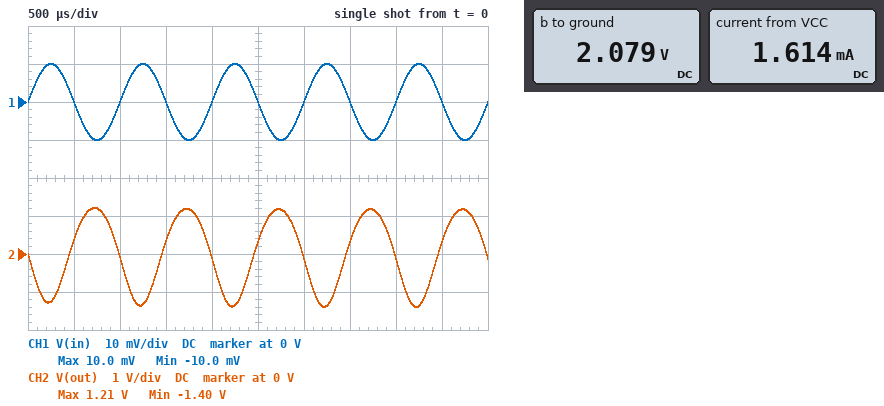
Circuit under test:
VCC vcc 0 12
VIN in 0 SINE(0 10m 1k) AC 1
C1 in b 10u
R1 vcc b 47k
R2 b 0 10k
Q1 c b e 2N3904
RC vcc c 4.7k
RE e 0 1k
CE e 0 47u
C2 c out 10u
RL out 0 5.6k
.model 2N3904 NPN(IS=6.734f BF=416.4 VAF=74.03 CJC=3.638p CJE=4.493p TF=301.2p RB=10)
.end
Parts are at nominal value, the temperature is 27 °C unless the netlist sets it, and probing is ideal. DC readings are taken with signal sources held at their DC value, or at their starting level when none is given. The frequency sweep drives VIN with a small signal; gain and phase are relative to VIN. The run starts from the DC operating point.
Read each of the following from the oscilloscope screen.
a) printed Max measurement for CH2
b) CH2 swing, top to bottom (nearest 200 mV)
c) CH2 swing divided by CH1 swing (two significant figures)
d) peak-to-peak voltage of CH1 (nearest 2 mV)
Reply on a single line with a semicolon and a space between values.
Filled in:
1.21 V; 2.6 V; 130; 20 mV
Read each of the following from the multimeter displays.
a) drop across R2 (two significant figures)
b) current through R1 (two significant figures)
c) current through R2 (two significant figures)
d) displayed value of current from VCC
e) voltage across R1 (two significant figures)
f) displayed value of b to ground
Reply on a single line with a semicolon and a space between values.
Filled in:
2.1 V; 210 µA; 210 µA; 1.614 mA; 9.9 V; 2.079 V
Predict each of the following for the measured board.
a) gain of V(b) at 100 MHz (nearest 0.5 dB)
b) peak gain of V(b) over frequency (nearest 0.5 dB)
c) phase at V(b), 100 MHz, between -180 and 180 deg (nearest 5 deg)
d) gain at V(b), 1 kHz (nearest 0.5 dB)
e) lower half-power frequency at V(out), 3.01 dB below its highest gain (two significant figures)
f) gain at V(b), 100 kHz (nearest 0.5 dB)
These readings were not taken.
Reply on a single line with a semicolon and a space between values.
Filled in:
0 dB; 0 dB; 0 deg; 0 dB; 180 Hz; 0 dB
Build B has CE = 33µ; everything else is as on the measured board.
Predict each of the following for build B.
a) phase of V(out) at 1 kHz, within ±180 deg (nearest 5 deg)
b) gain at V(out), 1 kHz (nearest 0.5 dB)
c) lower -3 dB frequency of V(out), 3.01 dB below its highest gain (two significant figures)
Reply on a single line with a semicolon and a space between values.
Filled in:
-165 deg; 42.0 dB; 260 Hz
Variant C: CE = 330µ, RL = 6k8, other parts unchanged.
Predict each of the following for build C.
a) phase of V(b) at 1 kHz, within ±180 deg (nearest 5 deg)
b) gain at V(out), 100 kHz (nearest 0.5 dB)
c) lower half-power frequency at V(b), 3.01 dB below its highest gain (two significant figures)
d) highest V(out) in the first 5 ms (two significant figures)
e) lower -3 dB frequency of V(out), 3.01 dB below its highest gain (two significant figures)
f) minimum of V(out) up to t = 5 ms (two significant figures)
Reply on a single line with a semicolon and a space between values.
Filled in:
0 deg; 43.0 dB; 2.2 Hz; 1.3 V; 28 Hz; -1.6 V
